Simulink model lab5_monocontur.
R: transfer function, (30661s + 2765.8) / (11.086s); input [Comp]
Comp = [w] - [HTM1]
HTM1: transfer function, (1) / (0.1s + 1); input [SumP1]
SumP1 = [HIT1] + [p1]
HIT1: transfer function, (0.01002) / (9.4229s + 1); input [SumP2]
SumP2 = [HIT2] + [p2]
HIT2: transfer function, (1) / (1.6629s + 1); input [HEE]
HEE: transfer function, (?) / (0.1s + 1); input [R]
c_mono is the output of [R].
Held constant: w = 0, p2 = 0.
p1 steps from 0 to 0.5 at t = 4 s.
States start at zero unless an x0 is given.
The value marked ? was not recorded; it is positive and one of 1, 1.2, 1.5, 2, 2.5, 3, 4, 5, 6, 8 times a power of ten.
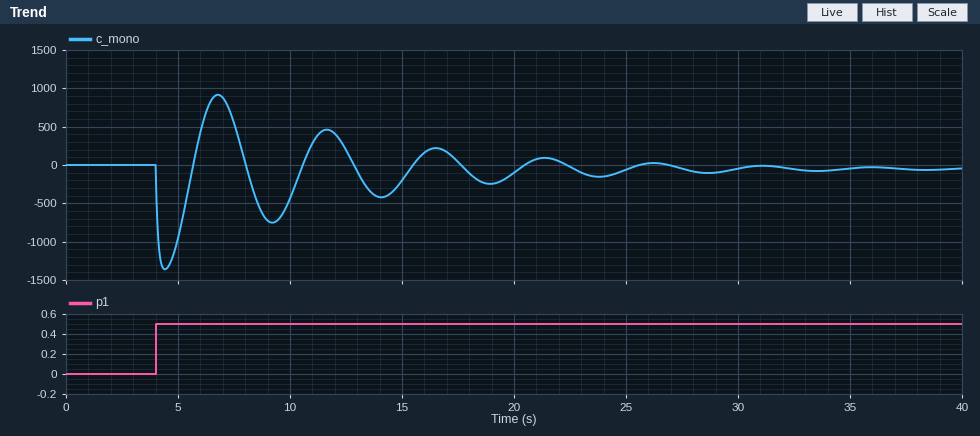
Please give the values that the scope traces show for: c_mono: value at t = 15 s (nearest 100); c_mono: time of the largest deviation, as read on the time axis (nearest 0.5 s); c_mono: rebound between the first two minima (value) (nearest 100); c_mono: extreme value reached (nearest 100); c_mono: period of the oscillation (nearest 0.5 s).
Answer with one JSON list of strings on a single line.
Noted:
["-200", "4.5 s", "900", "-1400", "5.0 s"]
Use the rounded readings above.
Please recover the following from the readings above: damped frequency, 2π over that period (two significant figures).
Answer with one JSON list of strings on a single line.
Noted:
["1.3 rad/s"]
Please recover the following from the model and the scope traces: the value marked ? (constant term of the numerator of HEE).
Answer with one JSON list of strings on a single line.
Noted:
["1"]
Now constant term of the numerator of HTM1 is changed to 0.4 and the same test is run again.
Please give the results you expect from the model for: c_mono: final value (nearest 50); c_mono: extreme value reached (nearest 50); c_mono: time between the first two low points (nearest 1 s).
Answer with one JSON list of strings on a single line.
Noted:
["-50", "-550", "8 s"]
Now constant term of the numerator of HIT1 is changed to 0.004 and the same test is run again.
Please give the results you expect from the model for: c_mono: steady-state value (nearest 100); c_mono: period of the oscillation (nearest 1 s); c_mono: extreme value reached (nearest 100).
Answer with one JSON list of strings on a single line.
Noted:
["-100", "8 s", "-1400"]
